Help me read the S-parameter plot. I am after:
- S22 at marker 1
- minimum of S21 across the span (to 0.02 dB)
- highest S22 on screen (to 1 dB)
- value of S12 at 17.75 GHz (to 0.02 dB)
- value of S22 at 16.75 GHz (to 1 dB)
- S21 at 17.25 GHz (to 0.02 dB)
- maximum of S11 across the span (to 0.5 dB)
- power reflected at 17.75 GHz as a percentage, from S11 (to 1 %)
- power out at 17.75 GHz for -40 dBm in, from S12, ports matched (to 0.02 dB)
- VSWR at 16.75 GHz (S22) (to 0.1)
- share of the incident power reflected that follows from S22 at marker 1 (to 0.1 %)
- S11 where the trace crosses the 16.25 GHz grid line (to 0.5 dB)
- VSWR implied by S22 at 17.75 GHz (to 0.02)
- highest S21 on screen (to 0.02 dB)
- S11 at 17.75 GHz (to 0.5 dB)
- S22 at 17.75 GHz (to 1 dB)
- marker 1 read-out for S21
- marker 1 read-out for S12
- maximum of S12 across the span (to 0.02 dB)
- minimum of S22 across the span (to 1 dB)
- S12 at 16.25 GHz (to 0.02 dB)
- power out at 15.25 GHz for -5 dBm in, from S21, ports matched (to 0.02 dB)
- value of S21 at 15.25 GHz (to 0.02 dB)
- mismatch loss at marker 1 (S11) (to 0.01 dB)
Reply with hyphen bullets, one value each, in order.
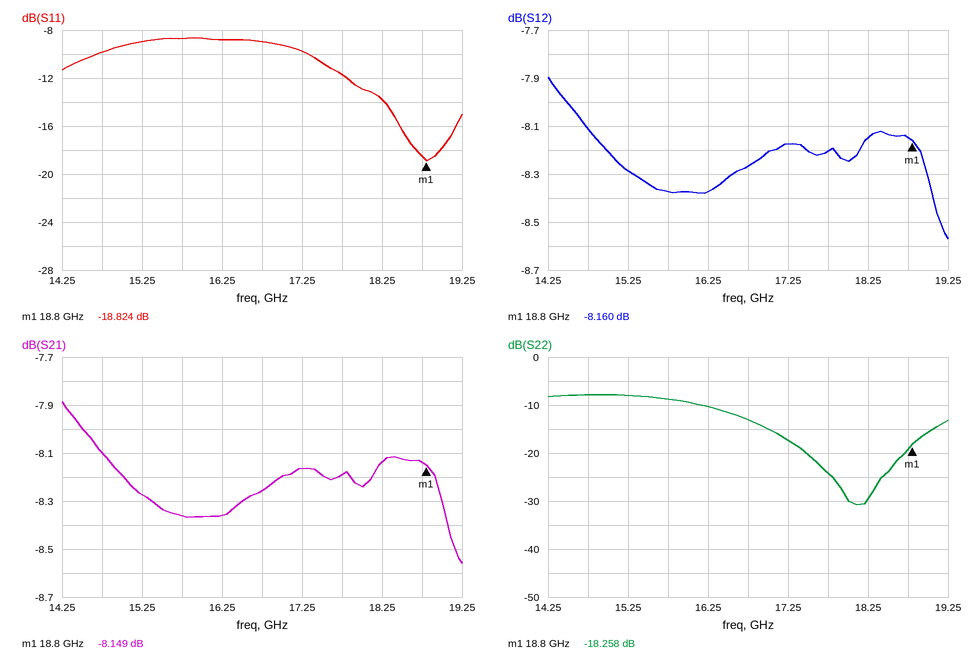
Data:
- -18.258 dB
- -8.56 dB
- -8 dB
- -8.20 dB
- -13 dB
- -8.16 dB
- -8.5 dB
- 7 %
- -48.20 dBm
- 1.6
- 1.5 %
- -9.0 dB
- 1.14
- -7.88 dB
- -11.5 dB
- -24 dB
- -8.149 dB
- -8.160 dB
- -7.90 dB
- -31 dB
- -8.38 dB
- -13.28 dBm
- -8.28 dB
- 0.06 dB
